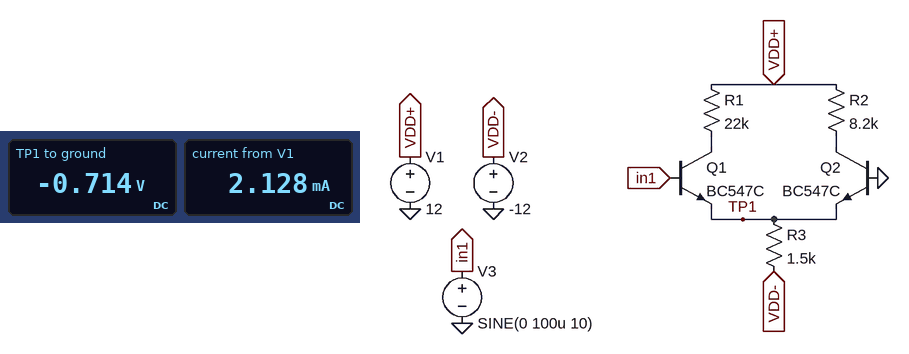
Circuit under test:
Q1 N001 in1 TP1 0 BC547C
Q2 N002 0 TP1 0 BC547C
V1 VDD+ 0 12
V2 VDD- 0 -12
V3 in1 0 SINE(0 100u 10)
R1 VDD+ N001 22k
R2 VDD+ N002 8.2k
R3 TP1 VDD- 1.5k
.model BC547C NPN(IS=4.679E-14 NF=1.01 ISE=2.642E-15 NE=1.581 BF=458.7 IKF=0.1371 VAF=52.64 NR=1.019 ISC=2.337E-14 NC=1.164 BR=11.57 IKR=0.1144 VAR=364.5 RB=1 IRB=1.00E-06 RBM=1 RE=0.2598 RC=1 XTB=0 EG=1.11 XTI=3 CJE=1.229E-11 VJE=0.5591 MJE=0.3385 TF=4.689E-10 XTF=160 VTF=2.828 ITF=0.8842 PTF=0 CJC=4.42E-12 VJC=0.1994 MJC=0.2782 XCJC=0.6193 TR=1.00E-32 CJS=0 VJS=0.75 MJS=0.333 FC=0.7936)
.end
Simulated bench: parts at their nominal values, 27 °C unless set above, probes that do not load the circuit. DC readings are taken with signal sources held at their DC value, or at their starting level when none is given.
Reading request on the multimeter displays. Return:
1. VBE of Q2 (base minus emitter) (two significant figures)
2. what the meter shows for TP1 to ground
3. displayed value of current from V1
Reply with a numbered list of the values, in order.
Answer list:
1. 710 mV
2. -0.714 V
3. 2.128 mA
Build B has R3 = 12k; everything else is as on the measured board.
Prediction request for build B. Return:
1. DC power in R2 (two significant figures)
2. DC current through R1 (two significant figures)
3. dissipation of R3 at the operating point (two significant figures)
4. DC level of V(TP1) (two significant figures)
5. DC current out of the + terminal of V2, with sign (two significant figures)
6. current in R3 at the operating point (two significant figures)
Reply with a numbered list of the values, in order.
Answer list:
1. 2.0 mW
2. 450 µA
3. 11 mW
4. -600 mV
5. -950 µA
6. 950 µA
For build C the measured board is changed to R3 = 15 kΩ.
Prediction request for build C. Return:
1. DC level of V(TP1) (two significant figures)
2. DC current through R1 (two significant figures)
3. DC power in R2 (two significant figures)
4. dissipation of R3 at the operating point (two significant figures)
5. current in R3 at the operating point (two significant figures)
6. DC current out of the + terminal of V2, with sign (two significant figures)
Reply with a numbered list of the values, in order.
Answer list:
1. -590 mV
2. 360 µA
3. 1.3 mW
4. 8.7 mW
5. 760 µA
6. -760 µA
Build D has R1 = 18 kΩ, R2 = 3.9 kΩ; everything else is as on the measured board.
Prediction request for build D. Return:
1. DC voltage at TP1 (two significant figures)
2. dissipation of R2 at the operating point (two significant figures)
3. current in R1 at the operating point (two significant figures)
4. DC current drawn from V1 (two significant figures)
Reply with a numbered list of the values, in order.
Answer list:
1. -700 mV
2. 41 mW
3. 710 µA
4. 4.0 mA
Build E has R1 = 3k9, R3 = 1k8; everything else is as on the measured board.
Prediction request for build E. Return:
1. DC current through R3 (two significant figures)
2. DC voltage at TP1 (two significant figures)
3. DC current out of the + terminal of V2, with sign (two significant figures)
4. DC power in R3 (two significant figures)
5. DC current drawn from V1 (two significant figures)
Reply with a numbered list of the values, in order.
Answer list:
1. 6.3 mA
2. -680 mV
3. -6.3 mA
4. 71 mW
5. 4.8 mA
